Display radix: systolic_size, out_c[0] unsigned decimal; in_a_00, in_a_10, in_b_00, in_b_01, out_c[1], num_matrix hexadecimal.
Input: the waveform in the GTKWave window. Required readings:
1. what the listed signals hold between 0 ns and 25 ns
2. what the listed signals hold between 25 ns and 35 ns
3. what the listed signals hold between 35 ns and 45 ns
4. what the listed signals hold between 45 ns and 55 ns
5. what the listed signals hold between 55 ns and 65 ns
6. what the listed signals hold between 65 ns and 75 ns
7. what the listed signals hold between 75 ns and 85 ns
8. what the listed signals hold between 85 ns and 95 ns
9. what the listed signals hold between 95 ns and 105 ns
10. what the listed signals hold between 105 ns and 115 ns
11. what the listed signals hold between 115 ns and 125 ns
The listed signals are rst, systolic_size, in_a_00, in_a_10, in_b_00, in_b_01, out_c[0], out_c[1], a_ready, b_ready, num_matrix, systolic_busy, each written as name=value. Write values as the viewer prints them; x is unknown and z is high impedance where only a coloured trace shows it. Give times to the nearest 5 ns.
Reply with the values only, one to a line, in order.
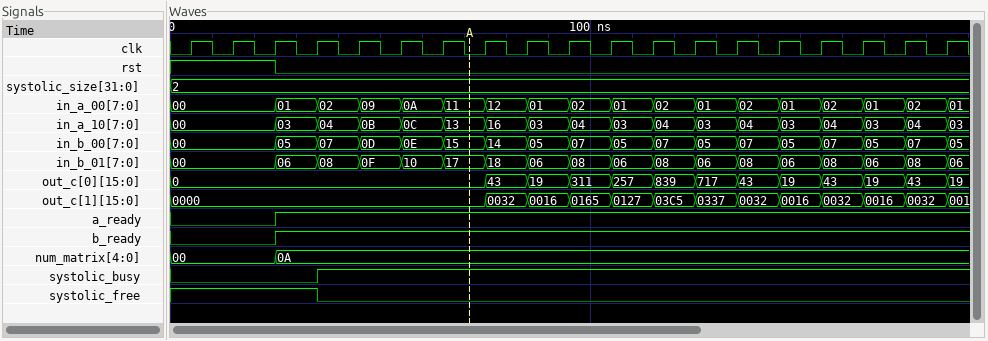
rst=1, systolic_size=2, in_a_00=00, in_a_10=00, in_b_00=00, in_b_01=00, out_c[0]=0, out_c[1]=0000, a_ready=0, b_ready=0, num_matrix=00, systolic_busy=0
rst=0, systolic_size=2, in_a_00=01, in_a_10=03, in_b_00=05, in_b_01=06, out_c[0]=0, out_c[1]=0000, a_ready=1, b_ready=1, num_matrix=0A, systolic_busy=0
rst=0, systolic_size=2, in_a_00=02, in_a_10=04, in_b_00=07, in_b_01=08, out_c[0]=0, out_c[1]=0000, a_ready=1, b_ready=1, num_matrix=0A, systolic_busy=1
rst=0, systolic_size=2, in_a_00=09, in_a_10=0B, in_b_00=0D, in_b_01=0F, out_c[0]=0, out_c[1]=0000, a_ready=1, b_ready=1, num_matrix=0A, systolic_busy=1
rst=0, systolic_size=2, in_a_00=0A, in_a_10=0C, in_b_00=0E, in_b_01=10, out_c[0]=0, out_c[1]=0000, a_ready=1, b_ready=1, num_matrix=0A, systolic_busy=1
rst=0, systolic_size=2, in_a_00=11, in_a_10=13, in_b_00=15, in_b_01=17, out_c[0]=0, out_c[1]=0000, a_ready=1, b_ready=1, num_matrix=0A, systolic_busy=1
rst=0, systolic_size=2, in_a_00=12, in_a_10=16, in_b_00=14, in_b_01=18, out_c[0]=43, out_c[1]=0032, a_ready=1, b_ready=1, num_matrix=0A, systolic_busy=1
rst=0, systolic_size=2, in_a_00=01, in_a_10=03, in_b_00=05, in_b_01=06, out_c[0]=19, out_c[1]=0016, a_ready=1, b_ready=1, num_matrix=0A, systolic_busy=1
rst=0, systolic_size=2, in_a_00=02, in_a_10=04, in_b_00=07, in_b_01=08, out_c[0]=311, out_c[1]=0165, a_ready=1, b_ready=1, num_matrix=0A, systolic_busy=1
rst=0, systolic_size=2, in_a_00=01, in_a_10=03, in_b_00=05, in_b_01=06, out_c[0]=257, out_c[1]=0127, a_ready=1, b_ready=1, num_matrix=0A, systolic_busy=1
rst=0, systolic_size=2, in_a_00=02, in_a_10=04, in_b_00=07, in_b_01=08, out_c[0]=839, out_c[1]=03C5, a_ready=1, b_ready=1, num_matrix=0A, systolic_busy=1
